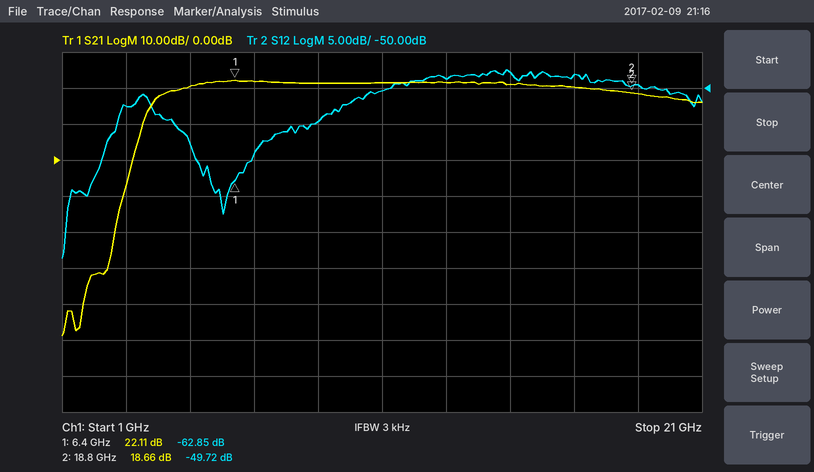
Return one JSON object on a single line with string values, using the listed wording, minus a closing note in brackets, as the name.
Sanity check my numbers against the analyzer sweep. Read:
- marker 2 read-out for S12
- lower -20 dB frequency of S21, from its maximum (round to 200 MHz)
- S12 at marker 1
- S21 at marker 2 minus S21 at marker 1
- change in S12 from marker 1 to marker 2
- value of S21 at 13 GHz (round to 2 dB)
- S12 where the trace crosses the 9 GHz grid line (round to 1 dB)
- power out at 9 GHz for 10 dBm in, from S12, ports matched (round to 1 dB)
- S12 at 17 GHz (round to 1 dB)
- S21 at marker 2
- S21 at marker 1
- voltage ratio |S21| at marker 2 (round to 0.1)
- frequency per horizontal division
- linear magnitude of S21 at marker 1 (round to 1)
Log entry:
{"marker 2 read-out for S12": "-49.72 dB", "lower -20 dB frequency of S21, from its maximum": "3.2 GHz", "S12 at marker 1": "-62.85 dB", "S21 at marker 2 minus S21 at marker 1": "-3.45 dB", "change in S12 from marker 1 to marker 2": "13.13 dB", "value of S21 at 13 GHz": "22 dB", "S12 where the trace crosses the 9 GHz grid line": "-55 dB", "power out at 9 GHz for 10 dBm in, from S12, ports matched": "-45 dBm", "S12 at 17 GHz": "-48 dB", "S21 at marker 2": "18.66 dB", "S21 at marker 1": "22.11 dB", "voltage ratio |S21| at marker 2": "8.6", "frequency per horizontal division": "2 GHz", "linear magnitude of S21 at marker 1": "13"}
